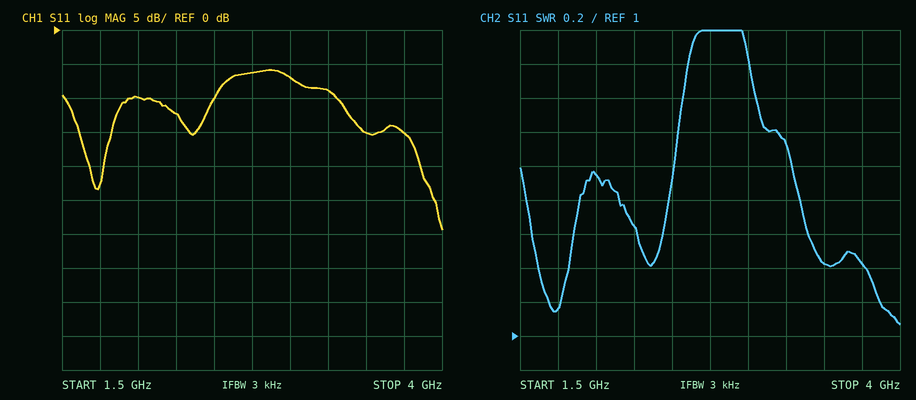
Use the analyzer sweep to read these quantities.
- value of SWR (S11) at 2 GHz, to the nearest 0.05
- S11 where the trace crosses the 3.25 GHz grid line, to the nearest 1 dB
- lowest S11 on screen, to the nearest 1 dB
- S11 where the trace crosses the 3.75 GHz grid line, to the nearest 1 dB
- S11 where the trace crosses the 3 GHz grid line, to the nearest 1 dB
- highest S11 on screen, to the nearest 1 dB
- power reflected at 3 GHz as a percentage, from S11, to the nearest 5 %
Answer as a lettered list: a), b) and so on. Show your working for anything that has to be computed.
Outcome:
a) 1.95
b) -9 dB
c) -29 dB
d) -15 dB
e) -7 dB
f) -6 dB
g) 10^(-7/10) ≈ 20 %
